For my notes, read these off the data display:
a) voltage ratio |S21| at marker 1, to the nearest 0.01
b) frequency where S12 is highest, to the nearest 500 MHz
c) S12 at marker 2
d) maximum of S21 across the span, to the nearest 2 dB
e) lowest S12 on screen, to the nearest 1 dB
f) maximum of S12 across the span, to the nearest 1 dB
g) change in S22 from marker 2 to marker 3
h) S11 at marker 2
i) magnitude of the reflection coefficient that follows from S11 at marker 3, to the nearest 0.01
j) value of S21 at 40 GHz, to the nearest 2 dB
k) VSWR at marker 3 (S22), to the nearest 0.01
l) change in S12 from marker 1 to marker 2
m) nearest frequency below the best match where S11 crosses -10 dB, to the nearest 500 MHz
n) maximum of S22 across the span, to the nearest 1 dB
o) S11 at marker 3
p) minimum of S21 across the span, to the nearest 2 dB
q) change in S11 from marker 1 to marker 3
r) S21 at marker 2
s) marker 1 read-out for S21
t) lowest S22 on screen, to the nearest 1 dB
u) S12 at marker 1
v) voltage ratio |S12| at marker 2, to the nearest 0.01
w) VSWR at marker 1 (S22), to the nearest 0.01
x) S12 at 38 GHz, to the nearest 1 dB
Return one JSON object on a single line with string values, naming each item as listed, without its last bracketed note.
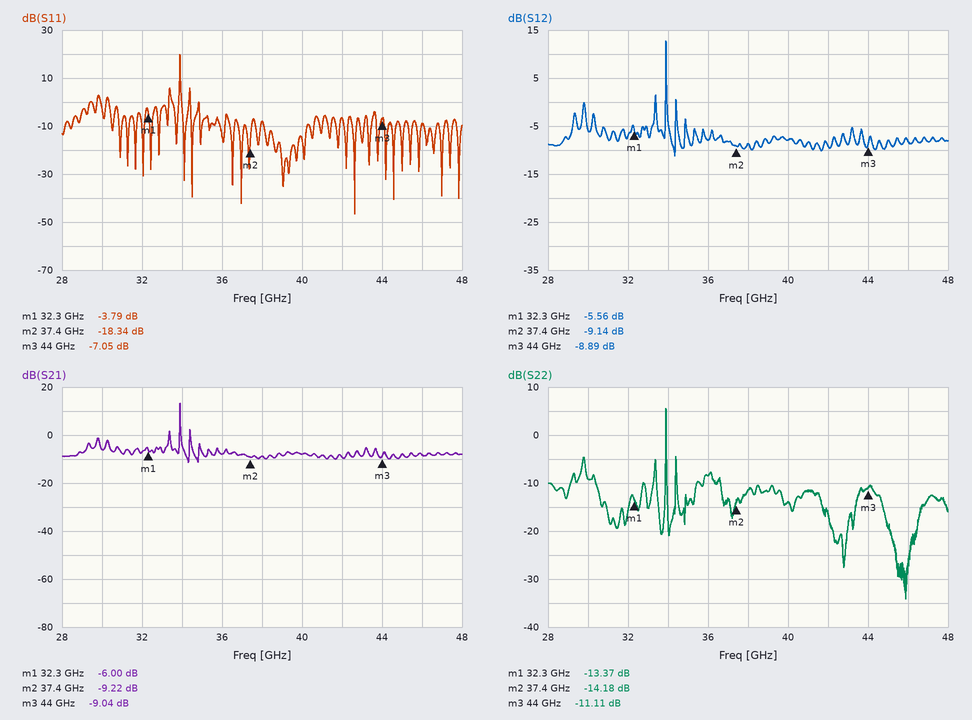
{"voltage ratio |S21| at marker 1, to the nearest 0.01": "0.50", "frequency where S12 is highest, to the nearest 500 MHz": "34.0 GHz", "S12 at marker 2": "-9.14 dB", "maximum of S21 across the span, to the nearest 2 dB": "14 dB", "lowest S12 on screen, to the nearest 1 dB": "-11 dB", "maximum of S12 across the span, to the nearest 1 dB": "13 dB", "change in S22 from marker 2 to marker 3": "3.07 dB", "S11 at marker 2": "-18.34 dB", "magnitude of the reflection coefficient that follows from S11 at marker 3, to the nearest 0.01": "0.44", "value of S21 at 40 GHz, to the nearest 2 dB": "-8 dB", "VSWR at marker 3 (S22), to the nearest 0.01": "1.77", "change in S12 from marker 1 to marker 2": "-3.58 dB", "nearest frequency below the best match where S11 crosses -10 dB, to the nearest 500 MHz": "42.5 GHz", "maximum of S22 across the span, to the nearest 1 dB": "6 dB", "S11 at marker 3": "-7.05 dB", "minimum of S21 across the span, to the nearest 2 dB": "-12 dB", "change in S11 from marker 1 to marker 3": "-3.26 dB", "S21 at marker 2": "-9.22 dB", "marker 1 read-out for S21": "-6.00 dB", "lowest S22 on screen, to the nearest 1 dB": "-34 dB", "S12 at marker 1": "-5.56 dB", "voltage ratio |S12| at marker 2, to the nearest 0.01": "0.35", "VSWR at marker 1 (S22), to the nearest 0.01": "1.55", "S12 at 38 GHz, to the nearest 1 dB": "-9 dB"}
